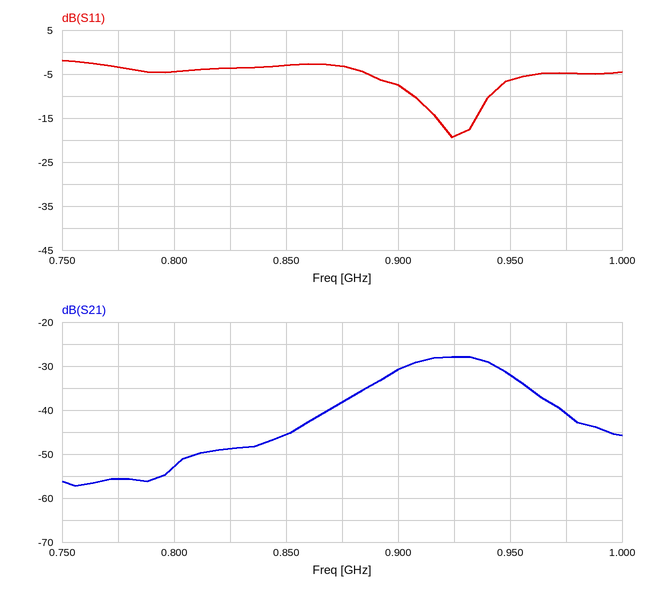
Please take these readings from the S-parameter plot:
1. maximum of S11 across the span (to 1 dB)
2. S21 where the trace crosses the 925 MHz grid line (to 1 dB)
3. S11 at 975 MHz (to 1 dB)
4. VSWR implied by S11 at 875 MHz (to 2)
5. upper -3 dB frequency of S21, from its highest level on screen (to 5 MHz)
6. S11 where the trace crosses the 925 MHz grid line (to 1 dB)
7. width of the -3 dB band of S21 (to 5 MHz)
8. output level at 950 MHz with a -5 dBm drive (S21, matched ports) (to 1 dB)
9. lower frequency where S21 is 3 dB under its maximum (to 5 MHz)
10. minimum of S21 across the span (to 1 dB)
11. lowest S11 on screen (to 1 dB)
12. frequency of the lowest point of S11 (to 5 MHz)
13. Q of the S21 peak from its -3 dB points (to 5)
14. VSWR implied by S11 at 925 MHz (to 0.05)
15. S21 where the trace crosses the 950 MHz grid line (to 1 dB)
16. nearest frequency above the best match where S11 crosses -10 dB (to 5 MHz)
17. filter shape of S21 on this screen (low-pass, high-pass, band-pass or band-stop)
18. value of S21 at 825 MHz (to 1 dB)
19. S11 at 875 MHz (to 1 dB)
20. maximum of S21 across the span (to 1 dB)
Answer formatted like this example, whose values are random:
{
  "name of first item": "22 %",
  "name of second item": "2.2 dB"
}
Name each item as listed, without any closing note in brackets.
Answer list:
{
  "maximum of S11 across the span": "-2 dB",
  "S21 where the trace crosses the 925 MHz grid line": "-28 dB",
  "S11 at 975 MHz": "-5 dB",
  "VSWR implied by S11 at 875 MHz": "6",
  "upper -3 dB frequency of S21, from its highest level on screen": "945 MHz",
  "S11 where the trace crosses the 925 MHz grid line": "-19 dB",
  "width of the -3 dB band of S21": "45 MHz",
  "output level at 950 MHz with a -5 dBm drive (S21, matched ports)": "-37 dBm",
  "lower frequency where S21 is 3 dB under its maximum": "900 MHz",
  "minimum of S21 across the span": "-57 dB",
  "lowest S11 on screen": "-19 dB",
  "frequency of the lowest point of S11": "925 MHz",
  "Q of the S21 peak from its -3 dB points": "20",
  "VSWR implied by S11 at 925 MHz": "1.25",
  "S21 where the trace crosses the 950 MHz grid line": "-32 dB",
  "nearest frequency above the best match where S11 crosses -10 dB": "940 MHz",
  "filter shape of S21 on this screen": "band-pass",
  "value of S21 at 825 MHz": "-49 dB",
  "S11 at 875 MHz": "-3 dB",
  "maximum of S21 across the span": "-28 dB"
}
